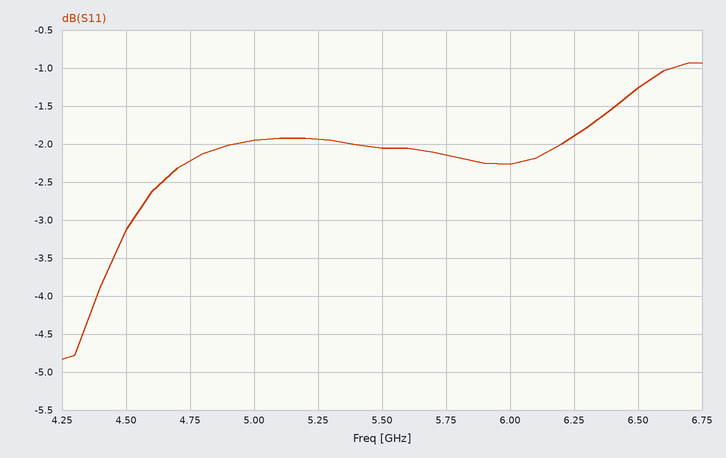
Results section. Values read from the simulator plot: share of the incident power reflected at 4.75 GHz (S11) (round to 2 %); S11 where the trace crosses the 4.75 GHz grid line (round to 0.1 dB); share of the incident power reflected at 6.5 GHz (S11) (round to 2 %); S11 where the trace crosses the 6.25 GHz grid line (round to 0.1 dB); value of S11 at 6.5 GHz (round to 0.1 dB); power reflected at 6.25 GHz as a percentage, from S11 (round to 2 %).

60 %
-2.2 dB
74 %
-1.9 dB
-1.3 dB
64 %
